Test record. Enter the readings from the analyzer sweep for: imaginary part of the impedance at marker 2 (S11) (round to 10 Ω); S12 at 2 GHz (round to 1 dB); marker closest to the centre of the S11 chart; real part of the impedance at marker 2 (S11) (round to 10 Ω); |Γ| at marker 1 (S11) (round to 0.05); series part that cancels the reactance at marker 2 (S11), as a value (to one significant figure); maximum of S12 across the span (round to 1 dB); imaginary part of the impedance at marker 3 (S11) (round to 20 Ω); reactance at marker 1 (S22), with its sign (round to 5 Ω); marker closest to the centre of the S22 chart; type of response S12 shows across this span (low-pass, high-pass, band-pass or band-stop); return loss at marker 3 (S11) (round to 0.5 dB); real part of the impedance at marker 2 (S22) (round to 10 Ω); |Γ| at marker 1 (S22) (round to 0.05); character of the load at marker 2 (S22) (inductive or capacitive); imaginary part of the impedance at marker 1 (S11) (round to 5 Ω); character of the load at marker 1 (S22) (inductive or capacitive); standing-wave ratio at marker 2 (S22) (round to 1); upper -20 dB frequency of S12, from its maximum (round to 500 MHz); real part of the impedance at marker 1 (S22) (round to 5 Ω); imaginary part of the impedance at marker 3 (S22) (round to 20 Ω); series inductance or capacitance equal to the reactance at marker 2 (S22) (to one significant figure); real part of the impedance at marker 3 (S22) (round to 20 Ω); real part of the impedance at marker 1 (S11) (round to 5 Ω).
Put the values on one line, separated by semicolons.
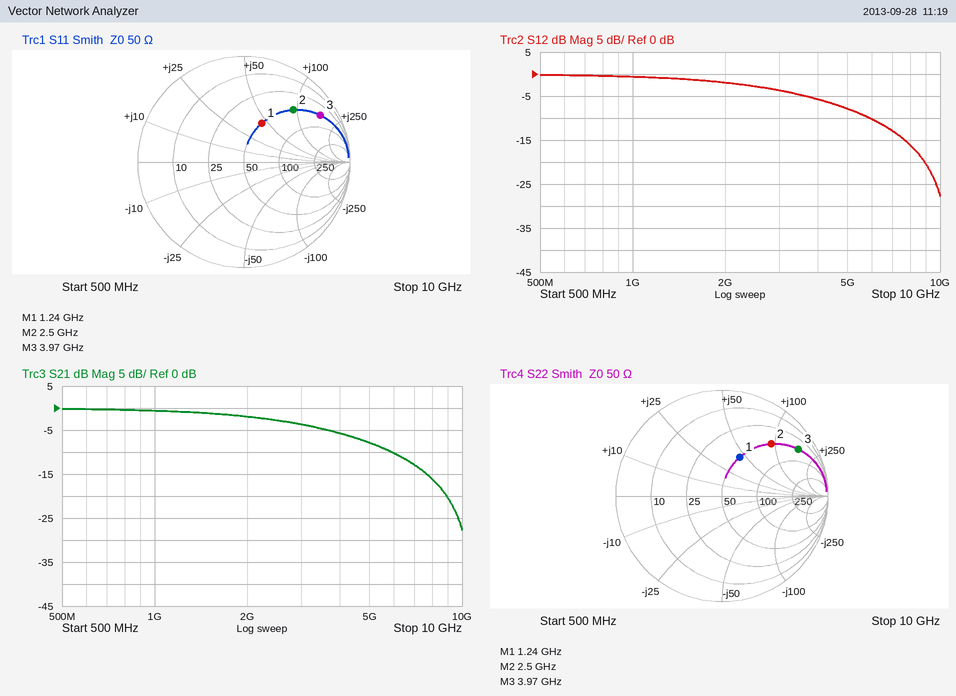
+90 Ω; -2 dB; marker 1; 50 Ω; 0.40; 700 fF; 0 dB; +160 Ω; +45 Ω; marker 1; low-pass; 1.5 dB; 50 Ω; 0.40; inductive; +45 Ω; inductive; 5; 9.0 GHz; 50 Ω; +160 Ω; 6 nH; 60 Ω; 50 Ω
